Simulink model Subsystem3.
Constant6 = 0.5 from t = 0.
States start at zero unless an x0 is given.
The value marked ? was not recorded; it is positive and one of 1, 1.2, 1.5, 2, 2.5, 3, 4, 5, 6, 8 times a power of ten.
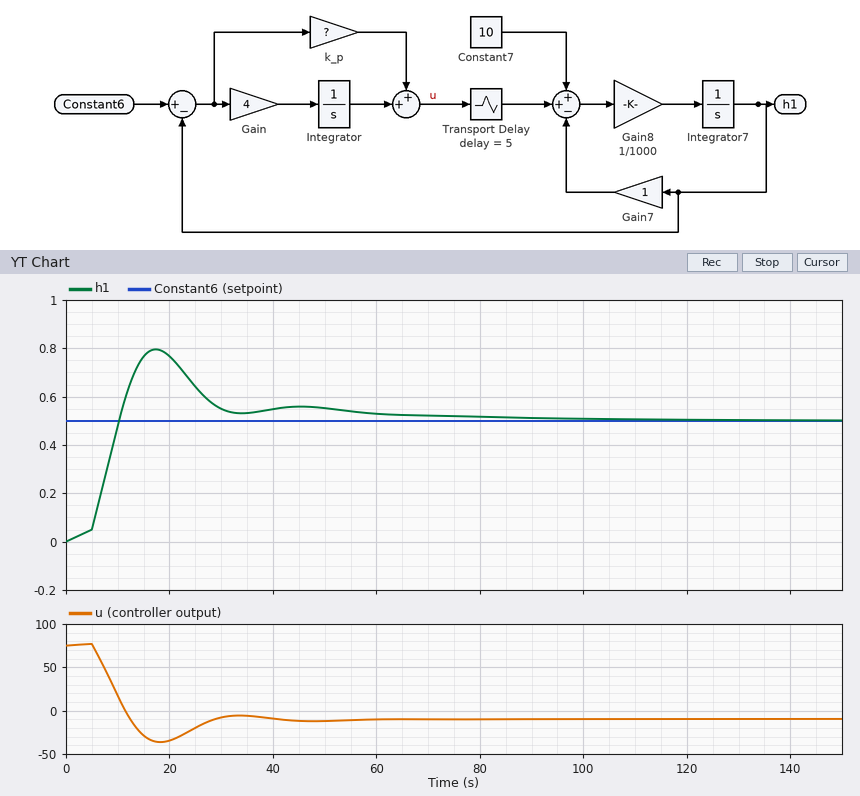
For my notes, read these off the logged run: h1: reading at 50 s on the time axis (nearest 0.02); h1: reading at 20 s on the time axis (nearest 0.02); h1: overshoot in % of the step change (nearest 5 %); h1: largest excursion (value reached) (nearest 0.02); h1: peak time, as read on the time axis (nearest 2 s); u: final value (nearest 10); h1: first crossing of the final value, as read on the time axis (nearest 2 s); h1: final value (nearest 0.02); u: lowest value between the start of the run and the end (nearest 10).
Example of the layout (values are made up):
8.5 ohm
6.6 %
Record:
0.56
0.76
60 %
0.80
18 s
-10
10 s
0.50
-40
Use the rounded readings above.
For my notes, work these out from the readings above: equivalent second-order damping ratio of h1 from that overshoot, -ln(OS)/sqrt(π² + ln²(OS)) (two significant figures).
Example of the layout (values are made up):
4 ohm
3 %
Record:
0.16
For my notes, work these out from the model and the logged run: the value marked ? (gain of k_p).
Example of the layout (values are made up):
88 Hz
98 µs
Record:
150
